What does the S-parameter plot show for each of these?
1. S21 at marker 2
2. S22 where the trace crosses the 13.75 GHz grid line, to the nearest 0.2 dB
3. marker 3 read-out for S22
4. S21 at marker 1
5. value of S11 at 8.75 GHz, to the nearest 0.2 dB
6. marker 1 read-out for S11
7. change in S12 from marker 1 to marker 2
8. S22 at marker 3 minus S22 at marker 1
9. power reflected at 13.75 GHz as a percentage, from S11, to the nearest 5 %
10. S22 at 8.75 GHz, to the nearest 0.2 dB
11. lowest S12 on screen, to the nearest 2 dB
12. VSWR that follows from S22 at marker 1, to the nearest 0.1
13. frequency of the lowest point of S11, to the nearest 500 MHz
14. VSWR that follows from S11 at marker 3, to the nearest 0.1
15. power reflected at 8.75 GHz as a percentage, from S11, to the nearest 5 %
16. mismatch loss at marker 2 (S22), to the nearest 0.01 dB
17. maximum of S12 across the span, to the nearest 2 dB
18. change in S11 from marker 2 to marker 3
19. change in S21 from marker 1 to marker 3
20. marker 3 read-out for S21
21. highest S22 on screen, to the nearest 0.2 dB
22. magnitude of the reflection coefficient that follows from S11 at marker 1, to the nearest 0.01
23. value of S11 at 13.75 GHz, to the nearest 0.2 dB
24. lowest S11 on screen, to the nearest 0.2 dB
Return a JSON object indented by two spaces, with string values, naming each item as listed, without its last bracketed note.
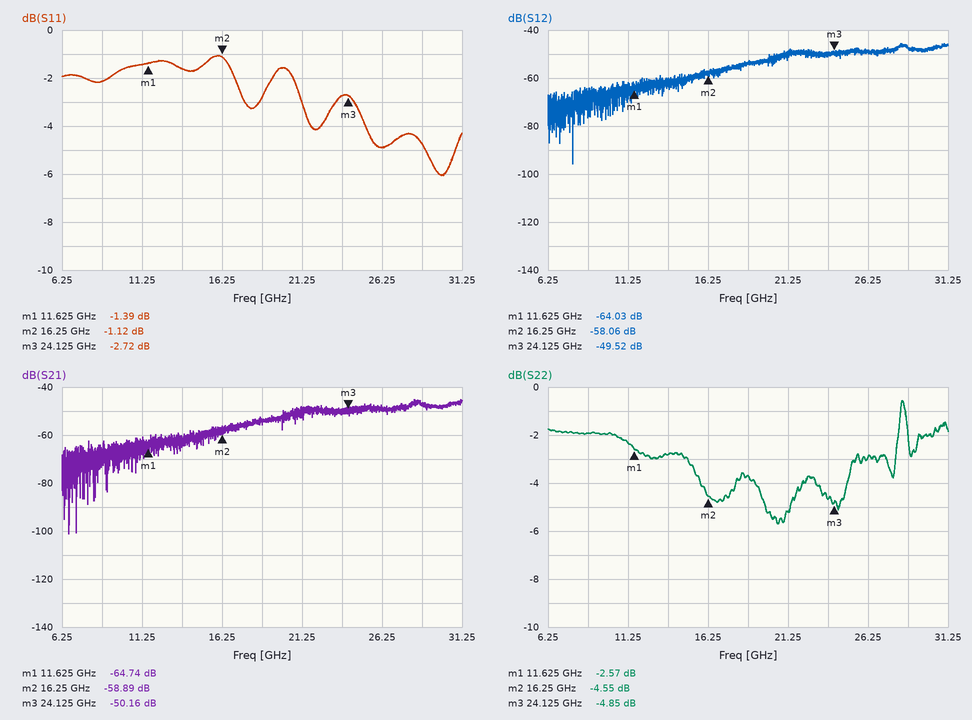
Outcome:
{
  "S21 at marker 2": "-58.89 dB",
  "S22 where the trace crosses the 13.75 GHz grid line, to the nearest 0.2 dB": "-2.8 dB",
  "marker 3 read-out for S22": "-4.85 dB",
  "S21 at marker 1": "-64.74 dB",
  "value of S11 at 8.75 GHz, to the nearest 0.2 dB": "-2.2 dB",
  "marker 1 read-out for S11": "-1.39 dB",
  "change in S12 from marker 1 to marker 2": "5.97 dB",
  "S22 at marker 3 minus S22 at marker 1": "-2.28 dB",
  "power reflected at 13.75 GHz as a percentage, from S11, to the nearest 5 %": "70 %",
  "S22 at 8.75 GHz, to the nearest 0.2 dB": "-2.0 dB",
  "lowest S12 on screen, to the nearest 2 dB": "-96 dB",
  "VSWR that follows from S22 at marker 1, to the nearest 0.1": "6.8",
  "frequency of the lowest point of S11, to the nearest 500 MHz": "30.0 GHz",
  "VSWR that follows from S11 at marker 3, to the nearest 0.1": "6.4",
  "power reflected at 8.75 GHz as a percentage, from S11, to the nearest 5 %": "60 %",
  "mismatch loss at marker 2 (S22), to the nearest 0.01 dB": "1.88 dB",
  "maximum of S12 across the span, to the nearest 2 dB": "-46 dB",
  "change in S11 from marker 2 to marker 3": "-1.60 dB",
  "change in S21 from marker 1 to marker 3": "14.58 dB",
  "marker 3 read-out for S21": "-50.16 dB",
  "highest S22 on screen, to the nearest 0.2 dB": "-0.6 dB",
  "magnitude of the reflection coefficient that follows from S11 at marker 1, to the nearest 0.01": "0.85",
  "value of S11 at 13.75 GHz, to the nearest 0.2 dB": "-1.6 dB",
  "lowest S11 on screen, to the nearest 0.2 dB": "-6.0 dB"
}
